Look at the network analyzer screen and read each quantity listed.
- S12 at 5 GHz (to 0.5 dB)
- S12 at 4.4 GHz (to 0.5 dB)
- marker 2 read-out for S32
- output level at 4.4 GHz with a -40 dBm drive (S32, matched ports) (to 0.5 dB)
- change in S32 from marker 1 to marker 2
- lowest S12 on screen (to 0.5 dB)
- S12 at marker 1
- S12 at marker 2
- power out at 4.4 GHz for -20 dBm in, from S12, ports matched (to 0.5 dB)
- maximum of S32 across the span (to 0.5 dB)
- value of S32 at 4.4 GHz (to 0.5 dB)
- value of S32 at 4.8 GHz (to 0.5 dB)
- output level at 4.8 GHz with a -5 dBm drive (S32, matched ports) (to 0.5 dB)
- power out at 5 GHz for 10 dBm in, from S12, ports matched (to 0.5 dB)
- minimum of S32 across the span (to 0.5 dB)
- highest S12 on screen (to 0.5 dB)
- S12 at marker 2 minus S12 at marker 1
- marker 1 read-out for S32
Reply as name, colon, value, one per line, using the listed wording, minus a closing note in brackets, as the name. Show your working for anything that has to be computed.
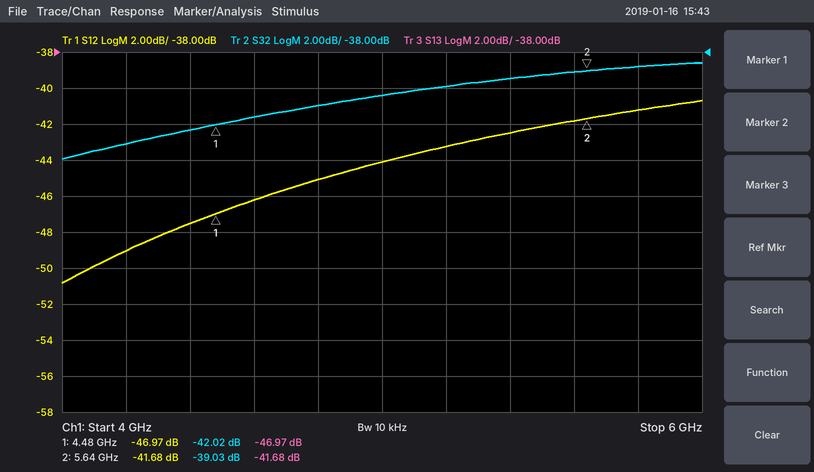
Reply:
S12 at 5 GHz: -44.0 dB
S12 at 4.4 GHz: -47.5 dB
marker 2 read-out for S32: -39.03 dB
output level at 4.4 GHz with a -40 dBm drive (S32, matched ports): -40 dBm + (-42.5 dB) = -82.5 dBm
change in S32 from marker 1 to marker 2: -39.03 − (-42.02) = 2.99 dB
lowest S12 on screen: -51.0 dB
S12 at marker 1: -46.97 dB
S12 at marker 2: -41.68 dB
power out at 4.4 GHz for -20 dBm in, from S12, ports matched: -20 dBm + (-47.5 dB) = -67.5 dBm
maximum of S32 across the span: -38.5 dB
value of S32 at 4.4 GHz: -42.5 dB
value of S32 at 4.8 GHz: -41.0 dB
output level at 4.8 GHz with a -5 dBm drive (S32, matched ports): -5 dBm + (-41.0 dB) = -46.0 dBm
power out at 5 GHz for 10 dBm in, from S12, ports matched: 10 dBm + (-44.0 dB) = -34.0 dBm
minimum of S32 across the span: -44.0 dB
highest S12 on screen: -40.5 dB
S12 at marker 2 minus S12 at marker 1: -41.68 − (-46.97) = 5.29 dB
marker 1 read-out for S32: -42.02 dB
